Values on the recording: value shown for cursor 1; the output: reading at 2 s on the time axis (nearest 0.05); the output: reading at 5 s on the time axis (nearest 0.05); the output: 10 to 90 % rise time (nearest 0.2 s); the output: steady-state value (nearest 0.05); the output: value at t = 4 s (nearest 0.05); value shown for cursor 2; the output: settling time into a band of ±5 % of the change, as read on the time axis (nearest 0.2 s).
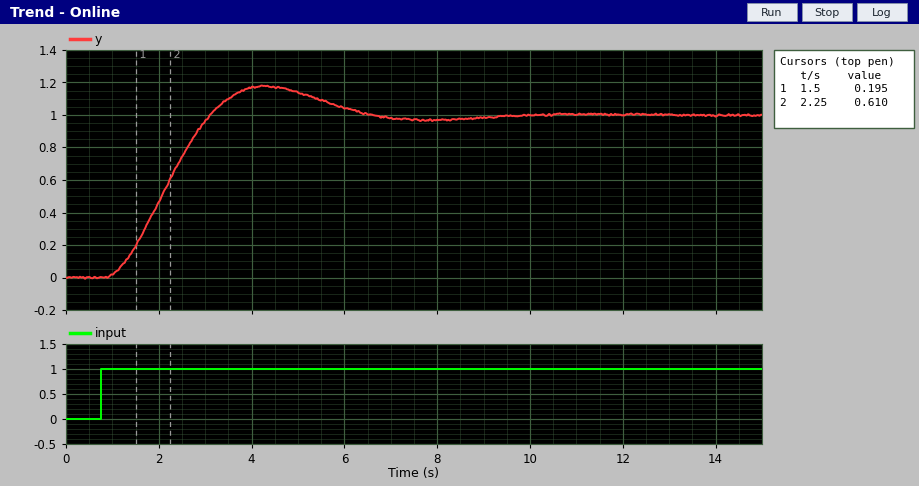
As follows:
0.195
0.45
1.15
1.6 s
1.00
1.15
0.610
6.0 s
